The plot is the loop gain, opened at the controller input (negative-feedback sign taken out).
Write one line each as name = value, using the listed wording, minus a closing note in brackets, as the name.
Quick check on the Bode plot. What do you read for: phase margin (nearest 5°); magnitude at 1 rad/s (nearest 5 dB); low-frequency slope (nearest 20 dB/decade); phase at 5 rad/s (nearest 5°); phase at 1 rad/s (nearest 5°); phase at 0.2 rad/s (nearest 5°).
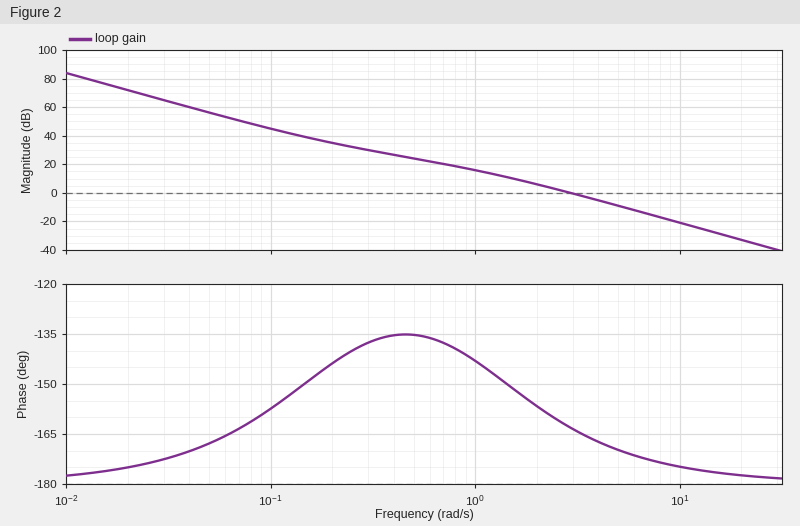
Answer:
phase margin = 15°
magnitude at 1 rad/s = 15 dB
low-frequency slope = -40 dB/decade
phase at 5 rad/s = -170°
phase at 1 rad/s = -145°
phase at 0.2 rad/s = -145°
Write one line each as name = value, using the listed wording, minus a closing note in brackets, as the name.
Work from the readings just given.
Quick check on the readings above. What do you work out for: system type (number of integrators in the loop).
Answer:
system type = 2
